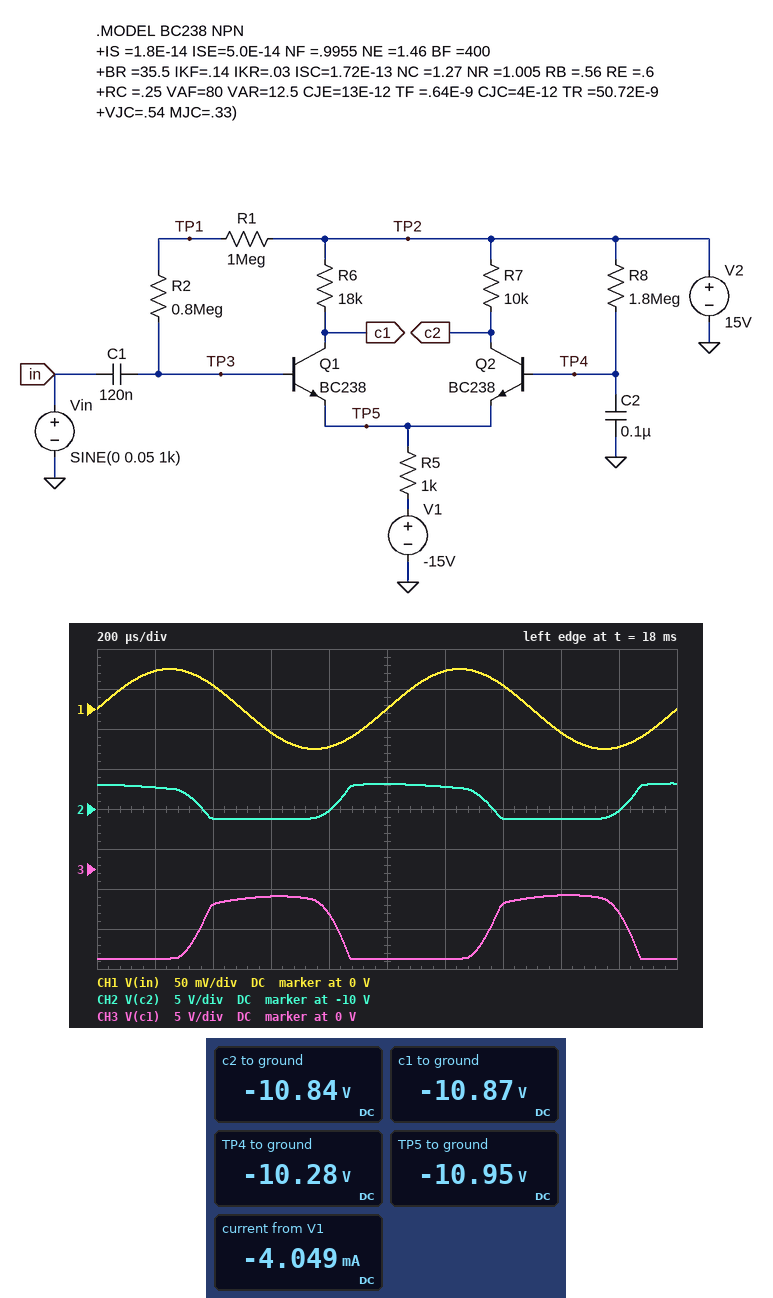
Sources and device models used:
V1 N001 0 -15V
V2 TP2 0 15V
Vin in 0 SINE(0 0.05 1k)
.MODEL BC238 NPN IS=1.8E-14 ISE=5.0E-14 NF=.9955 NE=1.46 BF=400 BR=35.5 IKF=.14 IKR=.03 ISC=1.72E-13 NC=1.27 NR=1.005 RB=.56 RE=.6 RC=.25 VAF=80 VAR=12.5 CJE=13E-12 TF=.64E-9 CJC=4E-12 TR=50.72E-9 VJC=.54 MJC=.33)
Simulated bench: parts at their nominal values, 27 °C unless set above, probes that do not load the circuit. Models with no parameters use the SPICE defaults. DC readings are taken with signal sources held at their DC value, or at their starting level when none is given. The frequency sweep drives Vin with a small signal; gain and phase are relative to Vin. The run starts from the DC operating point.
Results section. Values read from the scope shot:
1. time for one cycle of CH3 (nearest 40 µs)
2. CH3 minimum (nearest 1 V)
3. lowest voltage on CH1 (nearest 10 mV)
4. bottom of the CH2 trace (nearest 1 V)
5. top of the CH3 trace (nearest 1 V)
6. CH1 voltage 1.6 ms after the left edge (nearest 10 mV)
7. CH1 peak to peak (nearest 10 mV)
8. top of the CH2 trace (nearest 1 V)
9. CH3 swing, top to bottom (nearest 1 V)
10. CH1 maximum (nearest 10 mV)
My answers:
1.00 ms
-11 V
-50 mV
-11 V
-3 V
-30 mV
100 mV
-7 V
8 V
50 mV
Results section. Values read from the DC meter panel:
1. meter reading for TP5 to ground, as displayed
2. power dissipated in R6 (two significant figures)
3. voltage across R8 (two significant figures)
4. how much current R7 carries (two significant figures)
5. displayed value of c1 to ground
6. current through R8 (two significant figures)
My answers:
-10.95 V
37 mW
25 V
2.6 mA
-10.87 V
14 µA
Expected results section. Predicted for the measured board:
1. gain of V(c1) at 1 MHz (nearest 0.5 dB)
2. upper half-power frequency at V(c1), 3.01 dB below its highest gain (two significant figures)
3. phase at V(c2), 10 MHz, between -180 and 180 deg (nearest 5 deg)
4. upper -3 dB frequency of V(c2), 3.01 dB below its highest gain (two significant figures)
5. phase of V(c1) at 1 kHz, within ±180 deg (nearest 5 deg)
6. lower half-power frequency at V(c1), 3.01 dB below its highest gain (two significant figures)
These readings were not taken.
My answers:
20.5 dB
2.3 MHz
-70 deg
3.8 MHz
-105 deg
9.4 kHz
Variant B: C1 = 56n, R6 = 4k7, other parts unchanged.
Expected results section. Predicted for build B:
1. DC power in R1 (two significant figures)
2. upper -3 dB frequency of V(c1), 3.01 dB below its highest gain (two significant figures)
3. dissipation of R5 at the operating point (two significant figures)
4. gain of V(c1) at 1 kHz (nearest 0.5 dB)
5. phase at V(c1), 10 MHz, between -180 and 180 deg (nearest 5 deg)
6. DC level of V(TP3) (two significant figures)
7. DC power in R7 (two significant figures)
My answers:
160 µW
23 MHz
40 mW
17.0 dB
160 deg
-8.0 V
56 mW
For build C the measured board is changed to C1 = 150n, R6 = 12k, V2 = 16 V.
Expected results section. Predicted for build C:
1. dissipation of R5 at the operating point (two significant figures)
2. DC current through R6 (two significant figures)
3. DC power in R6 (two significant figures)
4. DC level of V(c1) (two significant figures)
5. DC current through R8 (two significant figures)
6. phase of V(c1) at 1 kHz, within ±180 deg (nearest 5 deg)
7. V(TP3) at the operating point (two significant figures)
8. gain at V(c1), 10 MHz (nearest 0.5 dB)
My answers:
23 mW
2.2 mA
57 mW
-10 V
14 µA
-110 deg
-9.5 V
16.0 dB
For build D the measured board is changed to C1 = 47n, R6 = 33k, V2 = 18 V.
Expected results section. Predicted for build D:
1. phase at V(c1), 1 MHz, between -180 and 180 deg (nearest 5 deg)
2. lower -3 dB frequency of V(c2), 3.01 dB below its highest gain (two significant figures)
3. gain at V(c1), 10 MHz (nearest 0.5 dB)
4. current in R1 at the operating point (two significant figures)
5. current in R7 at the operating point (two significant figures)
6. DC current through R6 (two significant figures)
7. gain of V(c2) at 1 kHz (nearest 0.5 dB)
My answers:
155 deg
42 kHz
5.5 dB
16 µA
2.9 mA
880 µA
-4.0 dB
